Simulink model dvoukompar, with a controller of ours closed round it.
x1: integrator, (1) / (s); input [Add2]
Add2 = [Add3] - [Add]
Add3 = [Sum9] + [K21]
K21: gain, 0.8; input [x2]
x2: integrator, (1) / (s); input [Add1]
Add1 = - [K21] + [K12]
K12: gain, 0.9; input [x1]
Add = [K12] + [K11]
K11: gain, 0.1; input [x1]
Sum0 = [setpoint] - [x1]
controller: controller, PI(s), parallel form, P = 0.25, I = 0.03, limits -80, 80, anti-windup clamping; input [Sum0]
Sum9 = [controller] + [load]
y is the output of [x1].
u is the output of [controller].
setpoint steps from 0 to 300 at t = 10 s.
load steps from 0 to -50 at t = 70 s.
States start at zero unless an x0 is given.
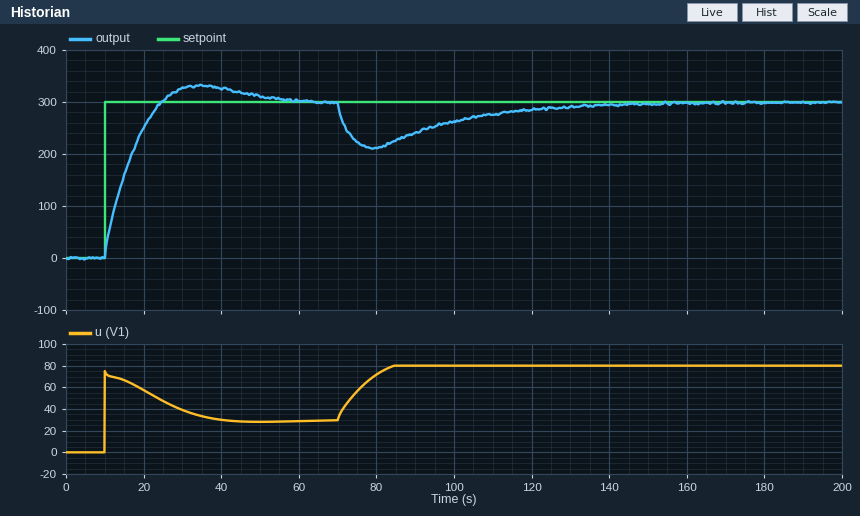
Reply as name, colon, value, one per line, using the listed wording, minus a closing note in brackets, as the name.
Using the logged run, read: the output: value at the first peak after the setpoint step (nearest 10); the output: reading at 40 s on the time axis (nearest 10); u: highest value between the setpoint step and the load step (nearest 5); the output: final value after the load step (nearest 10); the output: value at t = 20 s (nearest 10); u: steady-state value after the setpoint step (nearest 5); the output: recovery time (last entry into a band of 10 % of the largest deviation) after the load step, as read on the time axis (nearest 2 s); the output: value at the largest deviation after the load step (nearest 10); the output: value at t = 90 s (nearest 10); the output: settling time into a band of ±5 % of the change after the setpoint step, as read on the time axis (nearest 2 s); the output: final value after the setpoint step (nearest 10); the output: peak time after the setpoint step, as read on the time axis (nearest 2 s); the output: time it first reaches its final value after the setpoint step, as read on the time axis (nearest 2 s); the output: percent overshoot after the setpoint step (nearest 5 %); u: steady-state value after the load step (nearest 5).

the output: value at the first peak after the setpoint step: 330
the output: reading at 40 s on the time axis: 330
u: highest value between the setpoint step and the load step: 75
the output: final value after the load step: 300
the output: value at t = 20 s: 250
u: steady-state value after the setpoint step: 30
the output: recovery time (last entry into a band of 10 % of the largest deviation) after the load step, as read on the time axis: 132 s
the output: value at the largest deviation after the load step: 210
the output: value at t = 90 s: 240
the output: settling time into a band of ±5 % of the change after the setpoint step, as read on the time axis: 48 s
the output: final value after the setpoint step: 300
the output: peak time after the setpoint step, as read on the time axis: 34 s
the output: time it first reaches its final value after the setpoint step, as read on the time axis: 24 s
the output: percent overshoot after the setpoint step: 10 %
u: steady-state value after the load step: 80
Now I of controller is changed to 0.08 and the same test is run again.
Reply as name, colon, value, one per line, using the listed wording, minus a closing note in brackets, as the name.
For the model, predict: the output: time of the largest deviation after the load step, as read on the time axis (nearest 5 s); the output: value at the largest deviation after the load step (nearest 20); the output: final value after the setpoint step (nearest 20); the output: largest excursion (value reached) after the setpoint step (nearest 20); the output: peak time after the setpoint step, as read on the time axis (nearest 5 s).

the output: time of the largest deviation after the load step, as read on the time axis: 75 s
the output: value at the largest deviation after the load step: 240
the output: final value after the setpoint step: 300
the output: largest excursion (value reached) after the setpoint step: 360
the output: peak time after the setpoint step, as read on the time axis: 25 s
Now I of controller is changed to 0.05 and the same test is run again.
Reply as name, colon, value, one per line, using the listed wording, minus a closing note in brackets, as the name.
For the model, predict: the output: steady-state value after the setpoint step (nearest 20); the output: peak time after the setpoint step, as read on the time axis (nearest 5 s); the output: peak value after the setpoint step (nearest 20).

the output: steady-state value after the setpoint step: 300
the output: peak time after the setpoint step, as read on the time axis: 30 s
the output: peak value after the setpoint step: 360
